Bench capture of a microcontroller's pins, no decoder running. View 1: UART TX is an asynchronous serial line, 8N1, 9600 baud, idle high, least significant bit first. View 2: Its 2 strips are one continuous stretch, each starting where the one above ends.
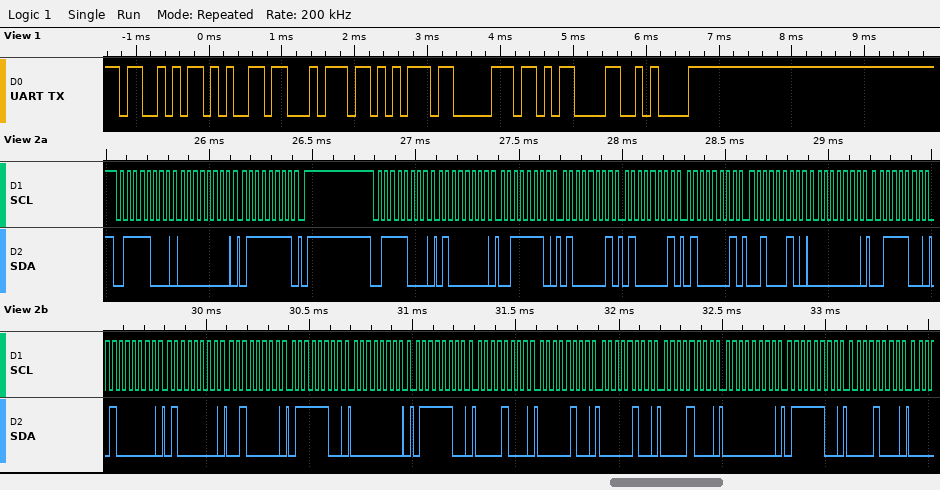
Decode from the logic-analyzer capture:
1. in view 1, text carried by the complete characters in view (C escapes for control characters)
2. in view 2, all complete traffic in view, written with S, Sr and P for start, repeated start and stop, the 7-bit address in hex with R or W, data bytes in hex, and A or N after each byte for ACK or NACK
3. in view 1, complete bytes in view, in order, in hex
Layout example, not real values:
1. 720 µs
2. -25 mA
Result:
1. "Setup\r\n"
2. S 3CW A 00 A 7F A P S 3CW A 40 A 3E A 41 A 41 A 41 A 22 A 00 A 3C A 40 A 40 A 20 A 7C A 00 A 7C A 08 A 04 A 04 A 08 A 00 A 7C A 08 A
3. 53 65 74 75 70 0D 0A
